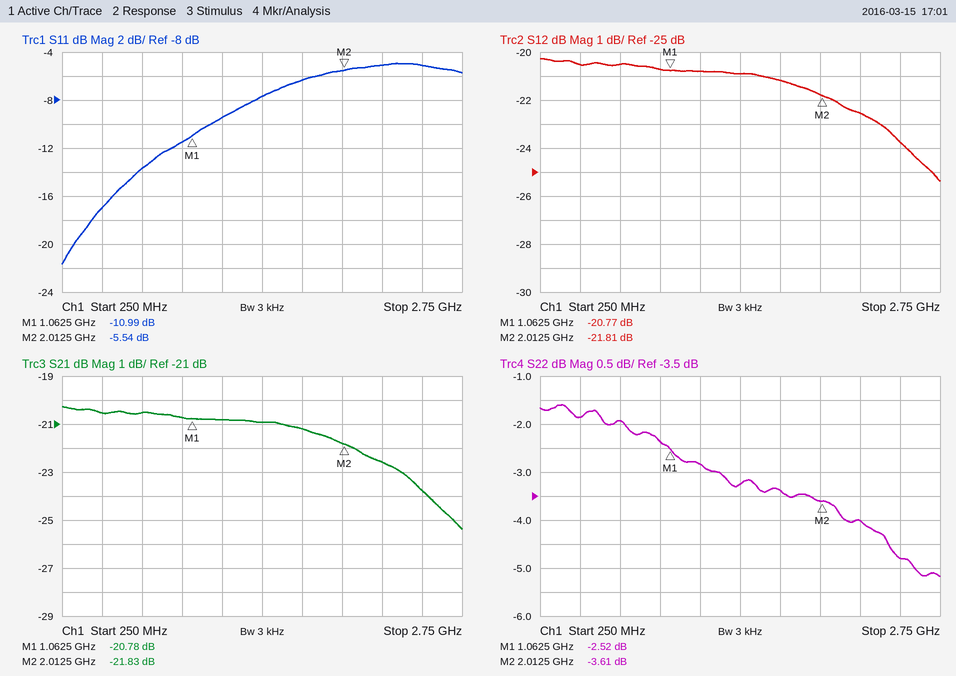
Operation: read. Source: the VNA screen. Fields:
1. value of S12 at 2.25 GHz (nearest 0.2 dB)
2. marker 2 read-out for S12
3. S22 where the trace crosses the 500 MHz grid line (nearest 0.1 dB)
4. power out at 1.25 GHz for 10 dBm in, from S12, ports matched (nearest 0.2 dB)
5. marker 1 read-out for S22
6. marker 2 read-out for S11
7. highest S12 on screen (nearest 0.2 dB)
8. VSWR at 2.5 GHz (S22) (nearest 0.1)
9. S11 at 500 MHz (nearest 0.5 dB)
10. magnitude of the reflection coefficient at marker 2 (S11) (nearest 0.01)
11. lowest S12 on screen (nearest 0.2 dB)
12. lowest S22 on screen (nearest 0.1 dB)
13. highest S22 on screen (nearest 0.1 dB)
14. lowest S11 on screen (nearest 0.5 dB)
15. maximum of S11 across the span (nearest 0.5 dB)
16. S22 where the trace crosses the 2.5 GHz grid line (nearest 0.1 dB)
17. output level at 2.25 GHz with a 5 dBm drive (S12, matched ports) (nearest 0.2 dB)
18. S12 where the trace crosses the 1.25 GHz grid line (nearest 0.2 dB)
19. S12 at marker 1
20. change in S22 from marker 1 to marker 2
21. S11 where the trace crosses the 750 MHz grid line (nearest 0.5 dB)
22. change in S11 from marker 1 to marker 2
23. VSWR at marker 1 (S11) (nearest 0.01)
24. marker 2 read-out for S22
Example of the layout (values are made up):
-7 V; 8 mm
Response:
-22.6 dB; -21.81 dB; -1.9 dB; -10.8 dBm; -2.52 dB; -5.54 dB; -20.2 dB; 3.7; -17.0 dB; 0.53; -25.4 dB; -5.2 dB; -1.6 dB; -21.5 dB; -5.0 dB; -4.8 dB; -17.6 dBm; -20.8 dB; -20.77 dB; -1.09 dB; -13.5 dB; 5.45 dB; 1.79; -3.61 dB
